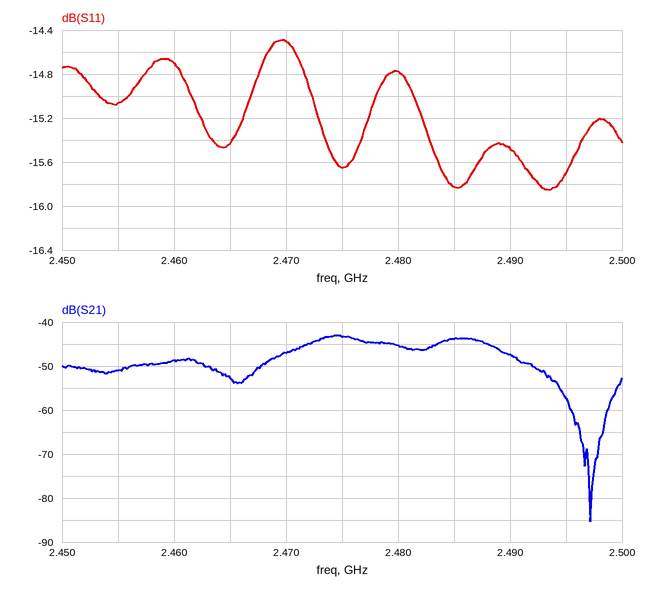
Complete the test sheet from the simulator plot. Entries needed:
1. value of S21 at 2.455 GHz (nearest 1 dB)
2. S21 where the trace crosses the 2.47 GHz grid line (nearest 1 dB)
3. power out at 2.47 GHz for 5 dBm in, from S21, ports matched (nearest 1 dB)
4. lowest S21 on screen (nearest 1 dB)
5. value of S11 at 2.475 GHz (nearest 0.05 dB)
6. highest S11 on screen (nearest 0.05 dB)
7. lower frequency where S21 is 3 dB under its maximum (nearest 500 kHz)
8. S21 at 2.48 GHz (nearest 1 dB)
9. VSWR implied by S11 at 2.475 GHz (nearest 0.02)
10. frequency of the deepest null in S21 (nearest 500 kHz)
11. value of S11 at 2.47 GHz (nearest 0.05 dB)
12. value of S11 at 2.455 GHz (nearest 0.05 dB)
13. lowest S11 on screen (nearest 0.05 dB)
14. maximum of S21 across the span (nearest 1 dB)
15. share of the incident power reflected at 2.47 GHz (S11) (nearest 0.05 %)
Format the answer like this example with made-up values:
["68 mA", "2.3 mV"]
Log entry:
["-51 dB", "-47 dB", "-42 dBm", "-85 dB", "-15.65 dB", "-14.50 dB", "2.4710 GHz", "-45 dB", "1.40", "2.4970 GHz", "-14.50 dB", "-15.05 dB", "-15.85 dB", "-43 dB", "3.55 %"]
